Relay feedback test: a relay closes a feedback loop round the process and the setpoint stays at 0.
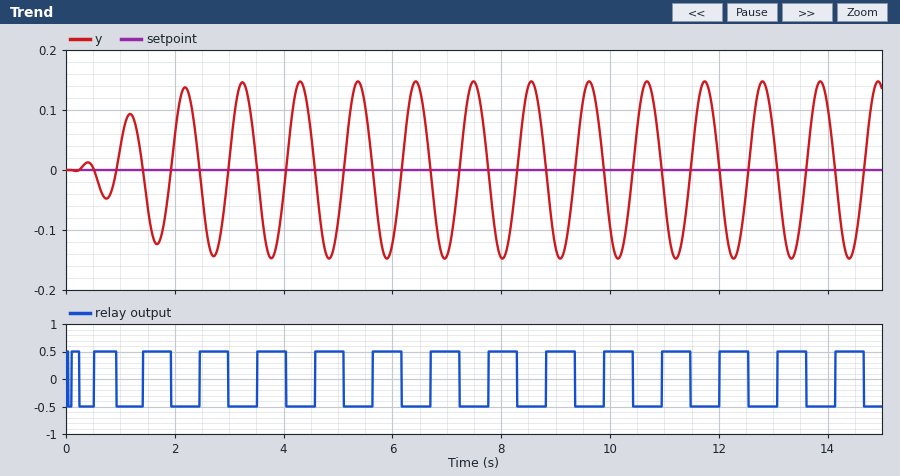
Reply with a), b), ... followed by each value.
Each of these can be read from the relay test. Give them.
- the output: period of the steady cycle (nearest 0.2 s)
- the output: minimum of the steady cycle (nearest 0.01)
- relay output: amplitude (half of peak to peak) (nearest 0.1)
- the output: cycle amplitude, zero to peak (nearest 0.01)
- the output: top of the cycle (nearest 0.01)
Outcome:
a) 1.0 s
b) -0.15
c) 0.5
d) 0.15
e) 0.15
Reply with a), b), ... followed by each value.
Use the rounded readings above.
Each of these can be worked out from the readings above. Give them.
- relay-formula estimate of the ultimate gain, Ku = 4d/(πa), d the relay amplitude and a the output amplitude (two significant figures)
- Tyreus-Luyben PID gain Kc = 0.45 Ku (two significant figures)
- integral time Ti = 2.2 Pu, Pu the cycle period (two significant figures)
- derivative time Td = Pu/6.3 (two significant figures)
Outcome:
a) 4.2
b) 1.9
c) 2.2 s
d) 0.16 s
